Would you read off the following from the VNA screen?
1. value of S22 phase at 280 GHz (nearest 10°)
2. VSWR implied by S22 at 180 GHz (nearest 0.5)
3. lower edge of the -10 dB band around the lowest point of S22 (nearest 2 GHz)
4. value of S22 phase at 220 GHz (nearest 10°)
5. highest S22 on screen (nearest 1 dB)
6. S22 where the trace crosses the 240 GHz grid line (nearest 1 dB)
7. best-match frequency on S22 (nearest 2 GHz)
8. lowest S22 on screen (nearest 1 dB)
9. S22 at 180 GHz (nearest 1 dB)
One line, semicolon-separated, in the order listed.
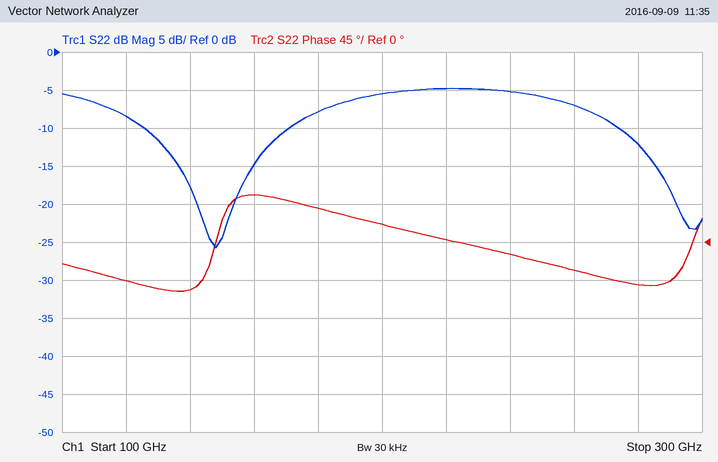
-50°; 2.5; 126 GHz; 0°; -5 dB; -5 dB; 148 GHz; -26 dB; -8 dB
